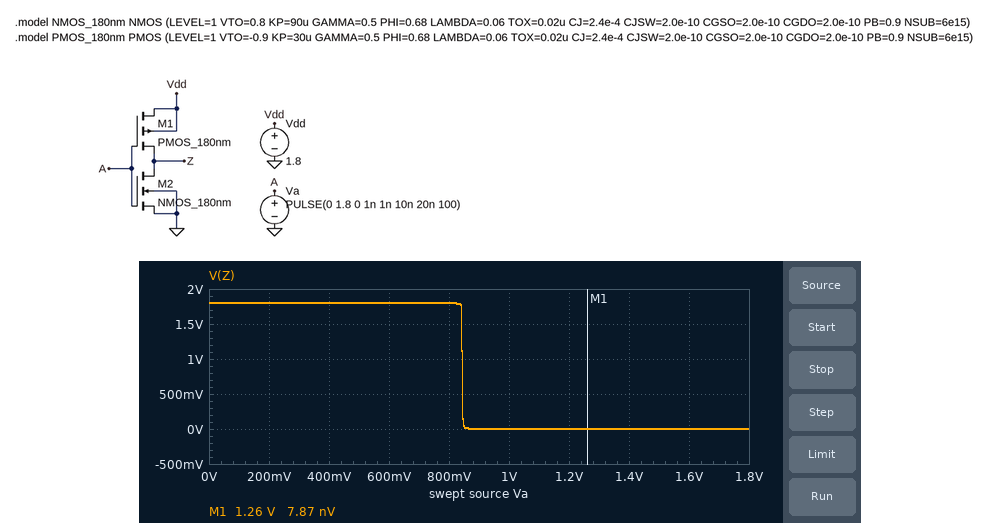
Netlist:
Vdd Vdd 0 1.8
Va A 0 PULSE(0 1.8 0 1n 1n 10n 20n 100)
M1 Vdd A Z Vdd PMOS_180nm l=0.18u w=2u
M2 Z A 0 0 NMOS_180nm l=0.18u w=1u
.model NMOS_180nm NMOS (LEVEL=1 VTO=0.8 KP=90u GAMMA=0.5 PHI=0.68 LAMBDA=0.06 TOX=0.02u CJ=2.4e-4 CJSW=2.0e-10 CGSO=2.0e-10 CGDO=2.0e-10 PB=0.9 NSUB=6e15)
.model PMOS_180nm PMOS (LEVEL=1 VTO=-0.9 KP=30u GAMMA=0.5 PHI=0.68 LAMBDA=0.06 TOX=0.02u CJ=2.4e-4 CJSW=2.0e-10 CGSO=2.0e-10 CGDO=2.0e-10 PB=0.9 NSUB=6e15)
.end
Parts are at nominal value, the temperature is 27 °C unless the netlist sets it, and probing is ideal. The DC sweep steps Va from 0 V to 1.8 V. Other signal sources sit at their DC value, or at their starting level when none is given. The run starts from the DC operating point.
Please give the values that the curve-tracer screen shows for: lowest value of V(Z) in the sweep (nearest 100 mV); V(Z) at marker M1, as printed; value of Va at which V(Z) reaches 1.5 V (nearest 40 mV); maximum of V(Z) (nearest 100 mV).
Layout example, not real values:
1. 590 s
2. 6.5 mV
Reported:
1. 0 V
2. 7.87 nV
3. 840 mV
4. 1.8 V
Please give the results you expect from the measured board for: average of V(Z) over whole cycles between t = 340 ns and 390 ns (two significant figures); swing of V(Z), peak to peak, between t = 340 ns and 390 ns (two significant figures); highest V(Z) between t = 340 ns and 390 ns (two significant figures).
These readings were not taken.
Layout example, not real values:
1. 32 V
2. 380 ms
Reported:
1. 800 mV
2. 1.9 V
3. 1.8 V
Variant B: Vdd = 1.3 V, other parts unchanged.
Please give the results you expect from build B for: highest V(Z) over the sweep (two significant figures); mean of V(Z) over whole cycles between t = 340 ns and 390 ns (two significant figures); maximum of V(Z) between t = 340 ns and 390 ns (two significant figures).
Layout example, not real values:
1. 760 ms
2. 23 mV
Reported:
1. 1.3 V
2. 560 mV
3. 1.7 V
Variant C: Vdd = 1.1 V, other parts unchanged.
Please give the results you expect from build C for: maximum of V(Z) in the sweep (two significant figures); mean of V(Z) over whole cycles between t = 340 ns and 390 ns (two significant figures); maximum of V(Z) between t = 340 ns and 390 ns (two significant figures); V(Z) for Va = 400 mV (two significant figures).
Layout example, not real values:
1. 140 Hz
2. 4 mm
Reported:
1. 1.1 V
2. 470 mV
3. 1.6 V
4. 550 mV
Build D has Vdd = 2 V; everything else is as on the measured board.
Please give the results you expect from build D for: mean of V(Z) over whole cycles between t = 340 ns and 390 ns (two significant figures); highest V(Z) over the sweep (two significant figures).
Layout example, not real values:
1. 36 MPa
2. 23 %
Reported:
1. 900 mV
2. 2.0 V
